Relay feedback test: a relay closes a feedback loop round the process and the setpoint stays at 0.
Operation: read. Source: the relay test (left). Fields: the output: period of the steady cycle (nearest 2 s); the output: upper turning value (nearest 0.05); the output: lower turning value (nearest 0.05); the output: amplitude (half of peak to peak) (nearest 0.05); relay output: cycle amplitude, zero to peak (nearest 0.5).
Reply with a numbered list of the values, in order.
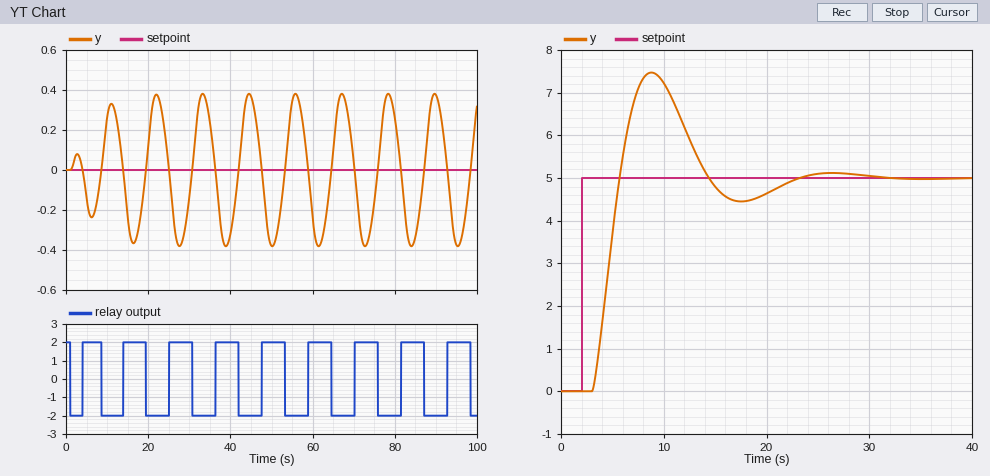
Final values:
1. 12 s
2. 0.40
3. -0.40
4. 0.40
5. 2.0
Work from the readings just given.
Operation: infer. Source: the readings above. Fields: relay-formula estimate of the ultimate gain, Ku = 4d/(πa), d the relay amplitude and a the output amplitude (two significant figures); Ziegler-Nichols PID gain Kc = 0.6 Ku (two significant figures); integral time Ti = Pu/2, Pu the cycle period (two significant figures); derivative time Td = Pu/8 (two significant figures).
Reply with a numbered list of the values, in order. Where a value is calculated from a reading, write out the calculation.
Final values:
1. 4 × 2 / (π × 0.4) = 6.4
2. 0.6 × 6.4 = 3.8
3. 12 / 2 = 6.0 s
4. 12 / 8 = 1.5 s
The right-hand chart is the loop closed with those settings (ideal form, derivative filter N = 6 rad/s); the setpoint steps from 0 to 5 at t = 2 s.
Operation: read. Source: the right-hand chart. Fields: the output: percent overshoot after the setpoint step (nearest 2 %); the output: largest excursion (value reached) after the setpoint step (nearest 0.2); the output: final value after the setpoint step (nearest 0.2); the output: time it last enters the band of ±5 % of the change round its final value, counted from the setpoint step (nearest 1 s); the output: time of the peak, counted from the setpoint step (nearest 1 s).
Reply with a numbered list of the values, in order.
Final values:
1. 50 %
2. 7.4
3. 5.0
4. 19 s
5. 7 s
